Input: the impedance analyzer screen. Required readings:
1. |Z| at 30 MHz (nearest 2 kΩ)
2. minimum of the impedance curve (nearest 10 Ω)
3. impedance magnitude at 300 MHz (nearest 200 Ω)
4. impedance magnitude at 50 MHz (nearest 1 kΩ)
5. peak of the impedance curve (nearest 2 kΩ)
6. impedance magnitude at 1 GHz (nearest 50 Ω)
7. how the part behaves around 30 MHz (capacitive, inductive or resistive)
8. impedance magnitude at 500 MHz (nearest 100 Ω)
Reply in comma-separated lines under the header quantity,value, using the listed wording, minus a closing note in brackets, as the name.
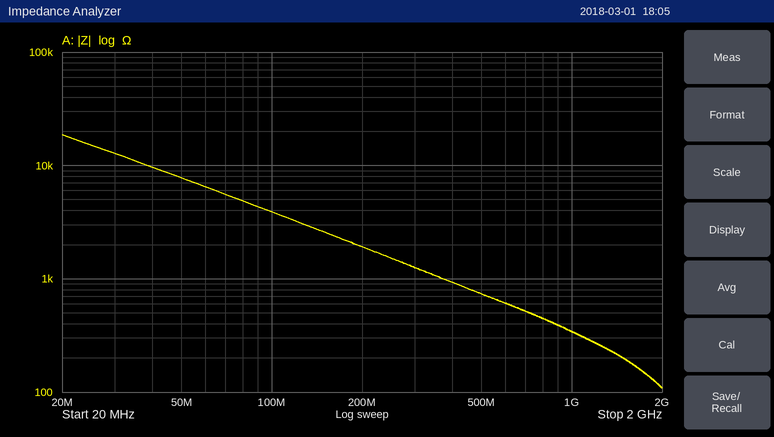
quantity,value
|Z| at 30 MHz,12 kΩ
minimum of the impedance curve,110 Ω
impedance magnitude at 300 MHz,1.2 kΩ
impedance magnitude at 50 MHz,8 kΩ
peak of the impedance curve,18 kΩ
impedance magnitude at 1 GHz,350 Ω
how the part behaves around 30 MHz,capacitive
impedance magnitude at 500 MHz,700 Ω
